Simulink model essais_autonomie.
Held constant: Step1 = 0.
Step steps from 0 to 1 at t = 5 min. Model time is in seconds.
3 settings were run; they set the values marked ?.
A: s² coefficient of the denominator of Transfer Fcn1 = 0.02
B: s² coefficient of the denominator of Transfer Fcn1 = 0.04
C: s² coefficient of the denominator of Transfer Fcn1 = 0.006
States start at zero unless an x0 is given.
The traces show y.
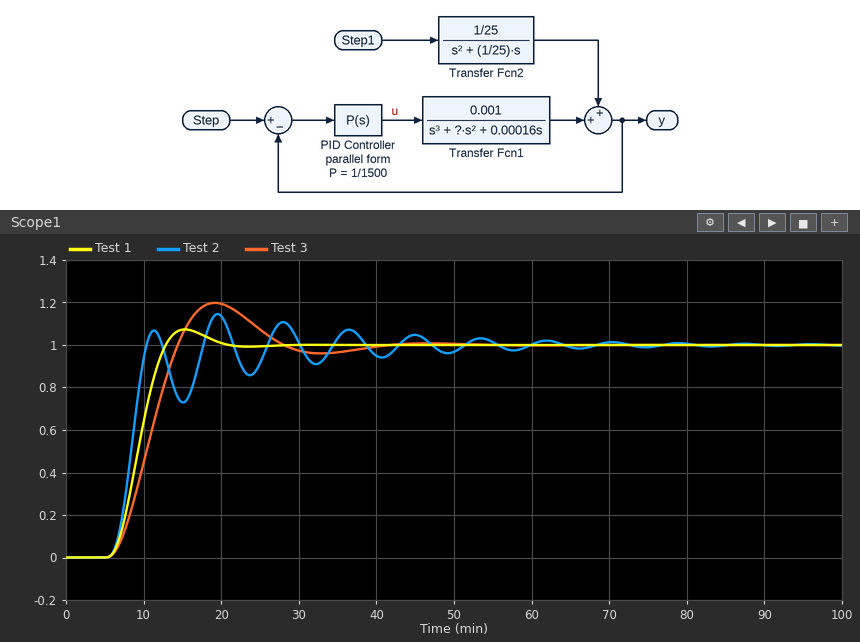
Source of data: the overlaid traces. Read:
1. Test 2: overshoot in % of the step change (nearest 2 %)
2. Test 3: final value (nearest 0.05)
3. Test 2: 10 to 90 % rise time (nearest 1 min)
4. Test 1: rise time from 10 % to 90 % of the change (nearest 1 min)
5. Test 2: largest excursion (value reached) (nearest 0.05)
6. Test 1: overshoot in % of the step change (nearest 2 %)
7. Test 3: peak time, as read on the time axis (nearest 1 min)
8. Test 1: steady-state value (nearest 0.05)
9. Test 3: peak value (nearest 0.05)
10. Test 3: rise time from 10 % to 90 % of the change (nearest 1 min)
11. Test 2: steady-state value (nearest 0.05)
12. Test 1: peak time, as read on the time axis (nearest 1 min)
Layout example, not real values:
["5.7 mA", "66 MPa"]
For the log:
["14 %", "1.00", "3 min", "5 min", "1.15", "8 %", "19 min", "1.00", "1.20", "6 min", "1.00", "15 min"]
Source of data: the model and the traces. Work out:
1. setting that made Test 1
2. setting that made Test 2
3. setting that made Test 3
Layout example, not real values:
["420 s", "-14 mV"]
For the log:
["A", "C", "B"]
